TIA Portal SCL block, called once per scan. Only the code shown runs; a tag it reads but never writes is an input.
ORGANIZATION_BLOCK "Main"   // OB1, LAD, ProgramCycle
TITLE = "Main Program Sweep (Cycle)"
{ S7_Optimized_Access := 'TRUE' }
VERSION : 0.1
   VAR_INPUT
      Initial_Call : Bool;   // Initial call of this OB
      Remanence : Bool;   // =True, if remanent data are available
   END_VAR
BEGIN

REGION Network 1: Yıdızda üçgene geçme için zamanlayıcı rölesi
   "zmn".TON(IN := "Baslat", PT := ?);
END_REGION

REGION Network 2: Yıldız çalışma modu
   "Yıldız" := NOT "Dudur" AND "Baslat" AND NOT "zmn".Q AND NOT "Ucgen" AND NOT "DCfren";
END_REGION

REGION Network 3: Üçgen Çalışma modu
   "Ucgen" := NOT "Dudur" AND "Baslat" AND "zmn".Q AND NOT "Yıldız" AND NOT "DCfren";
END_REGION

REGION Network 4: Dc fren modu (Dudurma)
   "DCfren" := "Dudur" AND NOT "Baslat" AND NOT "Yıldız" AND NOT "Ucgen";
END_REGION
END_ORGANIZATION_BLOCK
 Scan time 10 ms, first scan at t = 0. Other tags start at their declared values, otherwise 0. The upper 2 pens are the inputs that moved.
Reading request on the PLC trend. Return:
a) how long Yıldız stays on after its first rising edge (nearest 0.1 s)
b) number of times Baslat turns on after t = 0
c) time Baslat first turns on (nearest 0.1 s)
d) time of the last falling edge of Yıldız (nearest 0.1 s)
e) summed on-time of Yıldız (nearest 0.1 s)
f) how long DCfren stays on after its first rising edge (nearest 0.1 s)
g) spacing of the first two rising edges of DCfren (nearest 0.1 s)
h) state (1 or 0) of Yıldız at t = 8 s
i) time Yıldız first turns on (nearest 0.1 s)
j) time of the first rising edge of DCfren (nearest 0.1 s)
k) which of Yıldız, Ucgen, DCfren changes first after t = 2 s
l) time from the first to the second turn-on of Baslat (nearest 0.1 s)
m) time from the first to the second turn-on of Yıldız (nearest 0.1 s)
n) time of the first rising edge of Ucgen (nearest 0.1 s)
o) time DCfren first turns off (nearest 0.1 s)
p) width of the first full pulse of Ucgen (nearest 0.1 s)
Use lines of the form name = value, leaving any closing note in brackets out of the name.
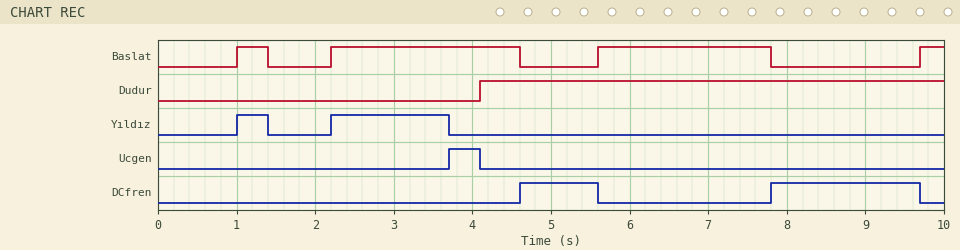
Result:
how long Yıldız stays on after its first rising edge = 0.4 s
number of times Baslat turns on after t = 0 = 4
time Baslat first turns on = 1.0 s
time of the last falling edge of Yıldız = 3.7 s
summed on-time of Yıldız = 1.9 s
how long DCfren stays on after its first rising edge = 1.0 s
spacing of the first two rising edges of DCfren = 3.2 s
state (1 or 0) of Yıldız at t = 8 s = 0
time Yıldız first turns on = 1.0 s
time of the first rising edge of DCfren = 4.6 s
which of Yıldız, Ucgen, DCfren changes first after t = 2 s = Yıldız
time from the first to the second turn-on of Baslat = 1.2 s
time from the first to the second turn-on of Yıldız = 1.2 s
time of the first rising edge of Ucgen = 3.7 s
time DCfren first turns off = 5.6 s
width of the first full pulse of Ucgen = 0.4 s
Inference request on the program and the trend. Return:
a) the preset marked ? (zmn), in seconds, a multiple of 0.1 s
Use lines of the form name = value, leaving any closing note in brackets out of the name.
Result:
the preset marked ? (zmn), in seconds, a multiple of 0.1 s = 1.5 s
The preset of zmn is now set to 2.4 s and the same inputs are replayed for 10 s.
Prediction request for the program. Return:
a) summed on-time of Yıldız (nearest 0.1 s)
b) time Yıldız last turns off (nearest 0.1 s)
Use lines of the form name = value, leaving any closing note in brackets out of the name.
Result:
summed on-time of Yıldız = 2.3 s
time Yıldız last turns off = 4.1 s
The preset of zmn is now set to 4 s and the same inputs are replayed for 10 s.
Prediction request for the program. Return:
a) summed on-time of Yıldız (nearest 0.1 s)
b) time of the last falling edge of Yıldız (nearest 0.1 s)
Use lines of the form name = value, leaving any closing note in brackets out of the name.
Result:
summed on-time of Yıldız = 2.3 s
time of the last falling edge of Yıldız = 4.1 s
